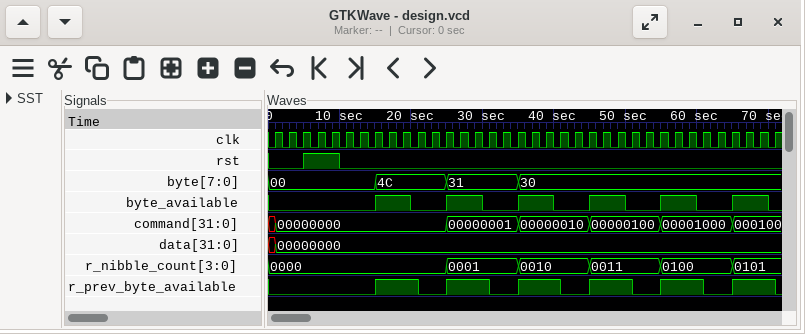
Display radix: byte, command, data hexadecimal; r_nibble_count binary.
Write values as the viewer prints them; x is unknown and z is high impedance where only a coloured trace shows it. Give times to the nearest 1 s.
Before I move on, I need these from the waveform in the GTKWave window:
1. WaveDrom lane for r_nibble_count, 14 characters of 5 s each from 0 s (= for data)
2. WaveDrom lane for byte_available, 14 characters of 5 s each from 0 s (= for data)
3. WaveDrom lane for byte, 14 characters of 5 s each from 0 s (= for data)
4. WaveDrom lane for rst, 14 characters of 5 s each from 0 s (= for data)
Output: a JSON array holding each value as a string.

["{name: 'r_nibble_count', wave: '=....=.=.=.=.=', data: '0000 0001 0010 0011 0100 0101'}", "{name: 'byte_available', wave: '0..10101010101'}", "{name: 'byte', wave: '=..=.=.=......', data: '00 4C 31 30'}", "{name: 'rst', wave: '010...........'}"]
